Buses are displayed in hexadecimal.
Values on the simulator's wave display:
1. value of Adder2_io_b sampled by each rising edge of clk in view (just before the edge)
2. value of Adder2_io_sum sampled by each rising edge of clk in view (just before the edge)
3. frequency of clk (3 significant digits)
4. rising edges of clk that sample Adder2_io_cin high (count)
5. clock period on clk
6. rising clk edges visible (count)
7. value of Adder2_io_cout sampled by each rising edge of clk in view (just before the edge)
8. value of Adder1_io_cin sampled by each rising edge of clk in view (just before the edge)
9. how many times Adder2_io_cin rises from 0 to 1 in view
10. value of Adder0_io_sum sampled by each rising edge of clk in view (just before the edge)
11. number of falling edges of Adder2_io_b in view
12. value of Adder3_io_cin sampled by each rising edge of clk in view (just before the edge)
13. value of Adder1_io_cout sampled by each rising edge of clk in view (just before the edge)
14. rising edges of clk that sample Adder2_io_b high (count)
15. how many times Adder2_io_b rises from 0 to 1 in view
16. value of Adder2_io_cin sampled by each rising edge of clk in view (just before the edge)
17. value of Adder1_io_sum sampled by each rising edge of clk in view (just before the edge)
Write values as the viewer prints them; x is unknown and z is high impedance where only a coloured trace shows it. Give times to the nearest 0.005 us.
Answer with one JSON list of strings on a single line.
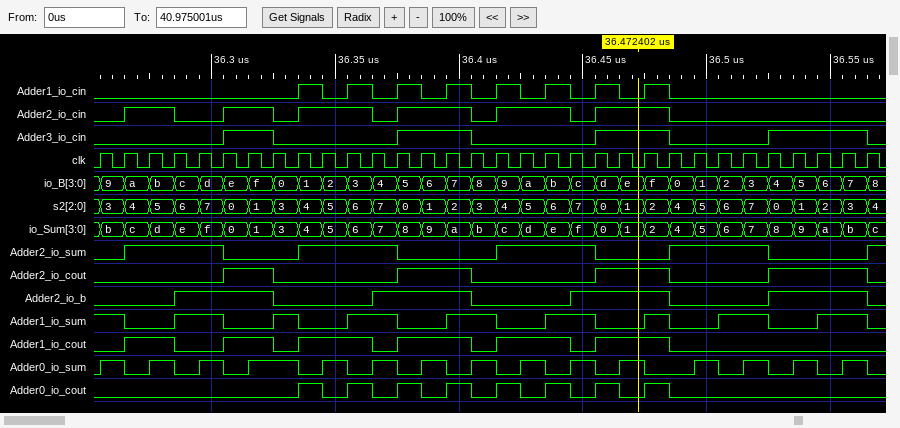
["0 0 0 0 1 1 1 1 0 0 0 0 1 1 1 1 0 0 0 0 1 1 1 1 0 0 0 0 1 1 1 1", "0 0 1 1 1 1 0 0 0 1 1 1 1 0 0 0 0 1 1 1 1 0 0 0 1 1 1 1 0 0 0 0", "100 MHz", "16", "0.01 us", "32", "0 0 0 0 0 0 1 1 0 0 0 0 0 1 1 1 0 0 0 0 0 1 1 1 0 0 0 0 1 1 1 1", "0 0 0 0 0 0 0 0 0 1 0 1 0 1 0 1 0 1 0 1 0 1 0 1 0 0 0 0 0 0 0 0", "6", "0 1 0 1 0 1 0 1 1 0 1 0 1 0 1 0 1 0 1 0 1 0 1 0 0 1 0 1 0 1 0 1", "4", "0 0 0 0 0 0 1 1 0 0 0 0 0 1 1 1 0 0 0 0 0 1 1 1 0 0 0 0 1 1 1 1", "0 0 1 1 0 0 1 1 0 1 1 1 0 1 1 1 0 1 1 1 0 1 1 1 0 0 0 0 0 0 0 0", "16", "4", "0 0 1 1 0 0 1 1 0 1 1 1 0 1 1 1 0 1 1 1 0 1 1 1 0 0 0 0 0 0 0 0", "1 1 0 0 1 1 0 0 1 0 0 1 1 0 0 1 1 0 0 1 1 0 0 1 0 0 1 1 0 0 1 1"]
